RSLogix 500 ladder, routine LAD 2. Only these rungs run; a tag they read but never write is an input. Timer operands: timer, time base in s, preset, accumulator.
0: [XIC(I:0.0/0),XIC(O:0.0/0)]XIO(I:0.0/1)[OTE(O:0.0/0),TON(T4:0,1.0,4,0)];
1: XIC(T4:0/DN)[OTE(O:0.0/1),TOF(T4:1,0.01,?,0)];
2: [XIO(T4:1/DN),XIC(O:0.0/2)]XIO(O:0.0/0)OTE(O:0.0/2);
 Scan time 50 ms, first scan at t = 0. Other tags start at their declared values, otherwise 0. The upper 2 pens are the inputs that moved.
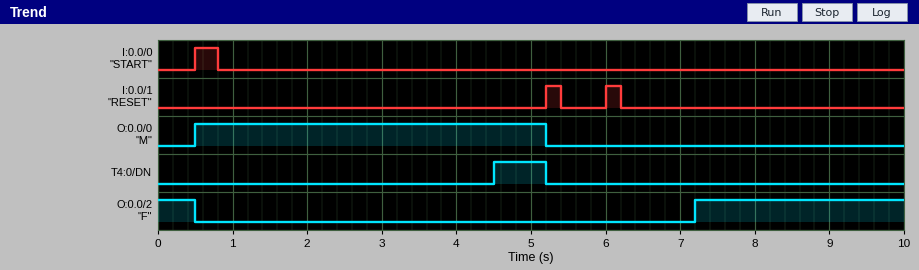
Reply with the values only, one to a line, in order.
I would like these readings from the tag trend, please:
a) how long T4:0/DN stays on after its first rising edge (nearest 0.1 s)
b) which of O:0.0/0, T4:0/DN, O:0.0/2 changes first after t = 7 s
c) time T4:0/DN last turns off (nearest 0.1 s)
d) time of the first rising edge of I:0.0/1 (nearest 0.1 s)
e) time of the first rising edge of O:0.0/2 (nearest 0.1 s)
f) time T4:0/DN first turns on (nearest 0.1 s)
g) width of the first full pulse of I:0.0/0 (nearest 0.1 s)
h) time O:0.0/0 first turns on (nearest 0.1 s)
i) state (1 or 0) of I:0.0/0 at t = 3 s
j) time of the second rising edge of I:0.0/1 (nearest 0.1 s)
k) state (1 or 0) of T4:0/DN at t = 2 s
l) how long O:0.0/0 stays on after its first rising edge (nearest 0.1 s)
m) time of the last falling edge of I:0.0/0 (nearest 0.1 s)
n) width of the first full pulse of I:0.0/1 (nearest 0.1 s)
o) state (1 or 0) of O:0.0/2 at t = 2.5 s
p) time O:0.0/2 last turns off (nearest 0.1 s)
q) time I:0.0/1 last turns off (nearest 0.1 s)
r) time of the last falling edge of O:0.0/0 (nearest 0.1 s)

0.7 s
O:0.0/2
5.2 s
5.2 s
7.2 s
4.5 s
0.3 s
0.5 s
0
6.0 s
0
4.7 s
0.8 s
0.2 s
0
0.5 s
6.2 s
5.2 s
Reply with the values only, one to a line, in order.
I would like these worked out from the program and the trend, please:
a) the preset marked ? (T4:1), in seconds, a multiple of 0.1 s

2.0 s
